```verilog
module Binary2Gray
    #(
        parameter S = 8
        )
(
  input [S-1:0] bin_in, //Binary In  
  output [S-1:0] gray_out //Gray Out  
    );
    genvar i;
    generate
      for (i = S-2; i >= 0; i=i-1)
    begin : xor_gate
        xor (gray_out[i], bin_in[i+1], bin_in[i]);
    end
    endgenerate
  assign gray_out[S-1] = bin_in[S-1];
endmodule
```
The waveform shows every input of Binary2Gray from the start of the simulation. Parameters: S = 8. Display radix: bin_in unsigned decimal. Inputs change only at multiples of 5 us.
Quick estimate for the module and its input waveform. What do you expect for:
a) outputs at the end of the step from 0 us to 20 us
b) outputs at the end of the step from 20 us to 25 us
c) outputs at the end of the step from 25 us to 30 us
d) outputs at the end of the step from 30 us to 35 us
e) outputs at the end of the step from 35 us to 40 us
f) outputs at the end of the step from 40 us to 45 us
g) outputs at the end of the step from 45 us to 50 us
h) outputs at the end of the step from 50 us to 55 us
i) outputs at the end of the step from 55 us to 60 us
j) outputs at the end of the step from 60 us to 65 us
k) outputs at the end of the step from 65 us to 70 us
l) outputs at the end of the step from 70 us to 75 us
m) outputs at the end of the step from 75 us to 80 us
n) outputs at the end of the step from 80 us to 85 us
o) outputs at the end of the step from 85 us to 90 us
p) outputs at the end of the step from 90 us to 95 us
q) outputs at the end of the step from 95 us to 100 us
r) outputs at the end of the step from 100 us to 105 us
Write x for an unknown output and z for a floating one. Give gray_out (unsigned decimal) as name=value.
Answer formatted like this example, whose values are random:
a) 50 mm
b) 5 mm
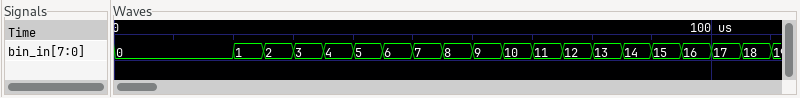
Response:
a) gray_out=0
b) gray_out=1
c) gray_out=3
d) gray_out=2
e) gray_out=6
f) gray_out=7
g) gray_out=5
h) gray_out=4
i) gray_out=12
j) gray_out=13
k) gray_out=15
l) gray_out=14
m) gray_out=10
n) gray_out=11
o) gray_out=9
p) gray_out=8
q) gray_out=24
r) gray_out=25
